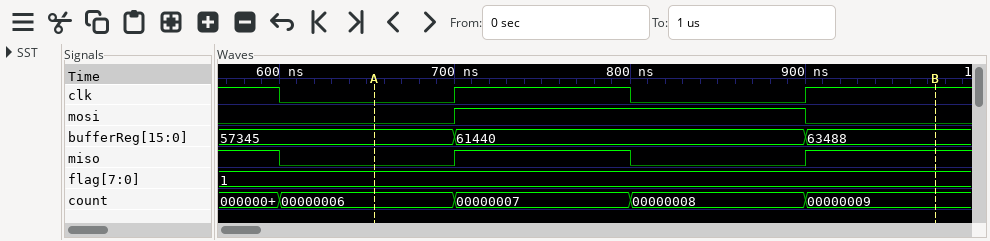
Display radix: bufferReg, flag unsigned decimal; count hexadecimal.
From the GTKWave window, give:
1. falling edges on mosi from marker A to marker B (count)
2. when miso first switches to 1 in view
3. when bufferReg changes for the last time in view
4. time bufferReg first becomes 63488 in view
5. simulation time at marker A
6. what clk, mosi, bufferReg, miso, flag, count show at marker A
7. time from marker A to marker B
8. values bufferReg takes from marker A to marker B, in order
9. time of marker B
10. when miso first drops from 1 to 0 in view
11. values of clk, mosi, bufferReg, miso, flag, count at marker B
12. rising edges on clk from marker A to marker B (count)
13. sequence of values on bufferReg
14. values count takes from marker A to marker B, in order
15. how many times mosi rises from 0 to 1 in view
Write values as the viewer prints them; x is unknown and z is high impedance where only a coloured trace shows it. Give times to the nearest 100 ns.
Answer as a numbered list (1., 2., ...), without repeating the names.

1. 1
2. 700 ns
3. 900 ns
4. 900 ns
5. 700 ns
6. clk=0, mosi=0, bufferReg=57345, miso=0, flag=1, count=00000006
7. 300 ns
8. 57345, 61440, 63488
9. 1000 ns
10. 600 ns
11. clk=1, mosi=0, bufferReg=63488, miso=1, flag=1, count=00000009
12. 2
13. 57345, 61440, 63488
14. 00000006, 00000007, 00000008, 00000009
15. 1
